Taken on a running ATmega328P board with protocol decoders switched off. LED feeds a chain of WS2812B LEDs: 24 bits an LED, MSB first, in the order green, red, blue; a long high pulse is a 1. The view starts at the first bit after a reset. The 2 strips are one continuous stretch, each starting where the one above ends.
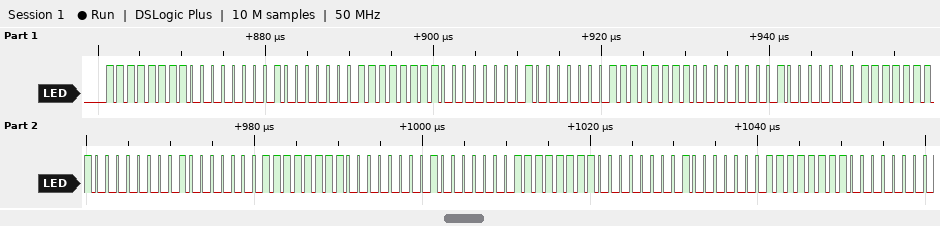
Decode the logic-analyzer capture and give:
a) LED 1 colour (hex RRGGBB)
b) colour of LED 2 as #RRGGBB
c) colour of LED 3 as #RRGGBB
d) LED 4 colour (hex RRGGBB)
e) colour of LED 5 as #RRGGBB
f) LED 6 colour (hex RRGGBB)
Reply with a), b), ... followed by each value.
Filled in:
a) #00FF80
b) #00FF80
c) #00FF80
d) #00FF80
e) #00FF80
f) #00FF80
